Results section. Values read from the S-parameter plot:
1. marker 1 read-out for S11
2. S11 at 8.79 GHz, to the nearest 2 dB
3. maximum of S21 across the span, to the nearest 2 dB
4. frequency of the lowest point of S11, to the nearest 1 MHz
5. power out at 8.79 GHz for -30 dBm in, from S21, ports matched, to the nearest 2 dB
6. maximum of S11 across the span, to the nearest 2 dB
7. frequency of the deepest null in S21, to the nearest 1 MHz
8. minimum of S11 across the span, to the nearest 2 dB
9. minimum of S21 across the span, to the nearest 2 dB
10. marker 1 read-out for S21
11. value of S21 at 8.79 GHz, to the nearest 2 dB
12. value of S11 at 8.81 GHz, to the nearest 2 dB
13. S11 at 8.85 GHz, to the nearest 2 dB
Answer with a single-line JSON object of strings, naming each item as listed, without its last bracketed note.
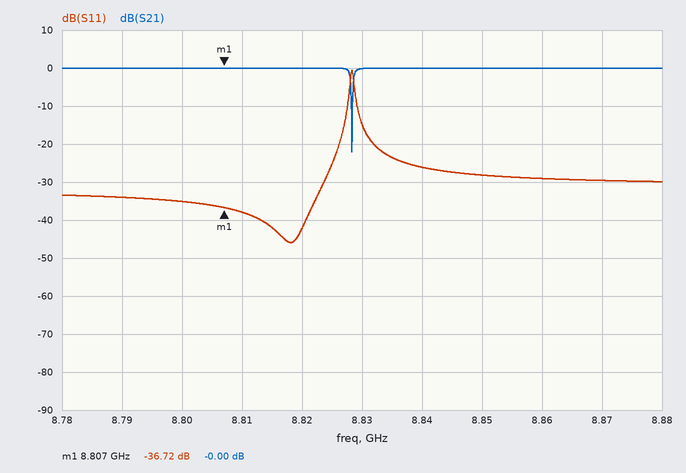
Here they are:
{"marker 1 read-out for S11": "-36.72 dB", "S11 at 8.79 GHz, to the nearest 2 dB": "-34 dB", "maximum of S21 across the span, to the nearest 2 dB": "0 dB", "frequency of the lowest point of S11, to the nearest 1 MHz": "8.818 GHz", "power out at 8.79 GHz for -30 dBm in, from S21, ports matched, to the nearest 2 dB": "-30 dBm", "maximum of S11 across the span, to the nearest 2 dB": "0 dB", "frequency of the deepest null in S21, to the nearest 1 MHz": "8.828 GHz", "minimum of S11 across the span, to the nearest 2 dB": "-46 dB", "minimum of S21 across the span, to the nearest 2 dB": "-22 dB", "marker 1 read-out for S21": "-0.00 dB", "value of S21 at 8.79 GHz, to the nearest 2 dB": "0 dB", "value of S11 at 8.81 GHz, to the nearest 2 dB": "-38 dB", "S11 at 8.85 GHz, to the nearest 2 dB": "-28 dB"}
